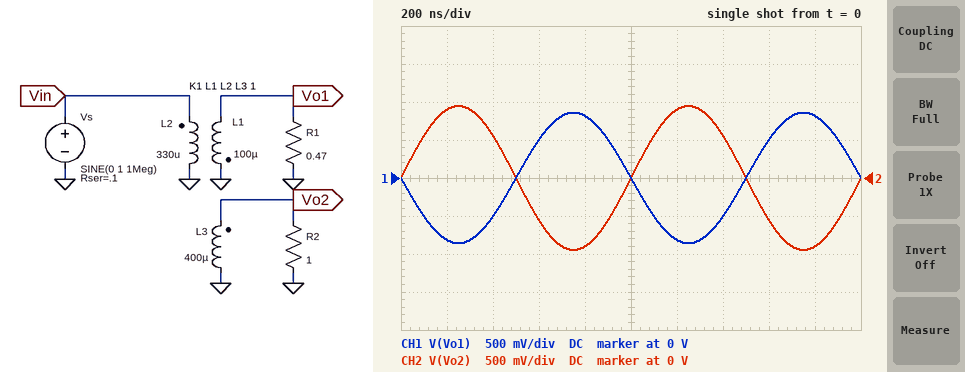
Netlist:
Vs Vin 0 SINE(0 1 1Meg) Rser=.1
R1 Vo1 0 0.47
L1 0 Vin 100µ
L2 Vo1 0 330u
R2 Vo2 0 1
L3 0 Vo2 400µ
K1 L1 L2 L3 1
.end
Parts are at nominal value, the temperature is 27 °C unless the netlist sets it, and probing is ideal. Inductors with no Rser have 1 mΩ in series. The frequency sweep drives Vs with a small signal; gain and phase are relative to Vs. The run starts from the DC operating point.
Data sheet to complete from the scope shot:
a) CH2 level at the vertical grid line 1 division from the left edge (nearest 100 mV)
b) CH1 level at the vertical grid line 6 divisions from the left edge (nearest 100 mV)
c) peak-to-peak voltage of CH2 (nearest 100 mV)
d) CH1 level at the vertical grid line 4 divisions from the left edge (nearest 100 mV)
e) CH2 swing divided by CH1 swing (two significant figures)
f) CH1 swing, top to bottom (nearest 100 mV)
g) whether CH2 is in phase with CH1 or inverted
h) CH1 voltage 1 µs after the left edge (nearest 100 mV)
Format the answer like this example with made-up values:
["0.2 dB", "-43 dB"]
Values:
["900 mV", "-800 mV", "1.9 V", "800 mV", "1.1", "1.7 V", "inverted", "0 V"]
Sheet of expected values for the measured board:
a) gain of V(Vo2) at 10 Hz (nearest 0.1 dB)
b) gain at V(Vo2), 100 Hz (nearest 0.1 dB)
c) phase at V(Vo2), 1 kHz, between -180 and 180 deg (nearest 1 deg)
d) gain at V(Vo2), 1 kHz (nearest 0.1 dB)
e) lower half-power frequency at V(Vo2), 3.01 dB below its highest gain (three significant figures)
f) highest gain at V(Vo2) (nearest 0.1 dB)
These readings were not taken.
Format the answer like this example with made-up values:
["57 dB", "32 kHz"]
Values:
["-18.2 dB", "-2.5 dB", "4 deg", "-0.5 dB", "76.1 Hz", "-0.5 dB"]
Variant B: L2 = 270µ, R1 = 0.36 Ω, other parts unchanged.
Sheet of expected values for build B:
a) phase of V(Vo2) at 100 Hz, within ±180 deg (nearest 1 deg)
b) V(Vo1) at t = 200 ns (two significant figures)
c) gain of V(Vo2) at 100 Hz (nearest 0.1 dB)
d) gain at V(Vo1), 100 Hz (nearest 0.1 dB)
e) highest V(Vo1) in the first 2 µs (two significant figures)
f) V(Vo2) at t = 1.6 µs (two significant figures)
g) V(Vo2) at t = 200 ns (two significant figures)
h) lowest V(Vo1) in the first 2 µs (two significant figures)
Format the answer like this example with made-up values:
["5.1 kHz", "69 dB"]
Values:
["37 deg", "-720 mV", "-2.6 dB", "-4.3 dB", "760 mV", "-540 mV", "880 mV", "-760 mV"]
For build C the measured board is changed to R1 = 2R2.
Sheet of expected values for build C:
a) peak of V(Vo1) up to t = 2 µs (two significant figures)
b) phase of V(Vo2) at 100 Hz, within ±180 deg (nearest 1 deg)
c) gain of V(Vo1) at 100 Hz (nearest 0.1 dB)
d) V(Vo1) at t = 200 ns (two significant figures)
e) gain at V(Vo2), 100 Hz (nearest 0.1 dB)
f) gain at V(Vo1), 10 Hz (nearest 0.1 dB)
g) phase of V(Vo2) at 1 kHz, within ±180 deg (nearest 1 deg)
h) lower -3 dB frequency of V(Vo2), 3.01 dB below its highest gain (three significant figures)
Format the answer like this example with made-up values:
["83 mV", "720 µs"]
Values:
["1.2 V", "46 deg", "-1.8 dB", "-1.1 V", "-1.0 dB", "-19.0 dB", "6 deg", "103 Hz"]
